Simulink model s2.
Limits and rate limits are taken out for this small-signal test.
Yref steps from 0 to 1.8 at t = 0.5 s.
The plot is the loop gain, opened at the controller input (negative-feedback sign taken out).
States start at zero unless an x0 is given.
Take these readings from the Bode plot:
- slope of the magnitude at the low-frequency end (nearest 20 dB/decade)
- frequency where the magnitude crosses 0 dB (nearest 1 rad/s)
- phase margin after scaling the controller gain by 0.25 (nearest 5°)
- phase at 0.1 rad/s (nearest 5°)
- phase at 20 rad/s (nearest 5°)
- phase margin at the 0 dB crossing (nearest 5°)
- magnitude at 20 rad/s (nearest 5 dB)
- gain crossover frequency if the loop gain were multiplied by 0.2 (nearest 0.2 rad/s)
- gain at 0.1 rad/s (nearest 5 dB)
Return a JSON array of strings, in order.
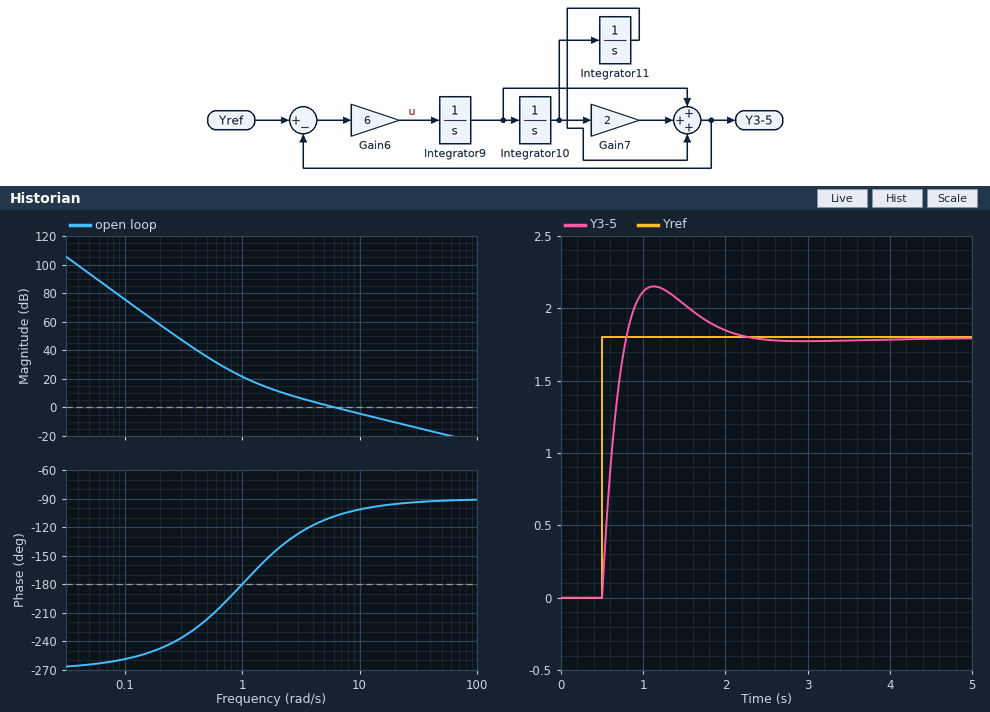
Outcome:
["-60 dB/decade", "6 rad/s", "35°", "-260°", "-95°", "70°", "-10 dB", "1.6 rad/s", "75 dB"]
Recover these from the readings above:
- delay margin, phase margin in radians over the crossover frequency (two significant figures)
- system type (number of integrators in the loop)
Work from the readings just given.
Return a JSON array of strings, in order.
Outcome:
["0.20 s", "3"]
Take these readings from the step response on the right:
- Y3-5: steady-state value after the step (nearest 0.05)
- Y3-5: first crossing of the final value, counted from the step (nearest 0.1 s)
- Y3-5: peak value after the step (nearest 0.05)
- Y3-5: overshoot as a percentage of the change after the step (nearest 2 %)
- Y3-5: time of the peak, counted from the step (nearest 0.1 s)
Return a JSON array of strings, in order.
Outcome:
["1.80", "0.3 s", "2.15", "20 %", "0.6 s"]
